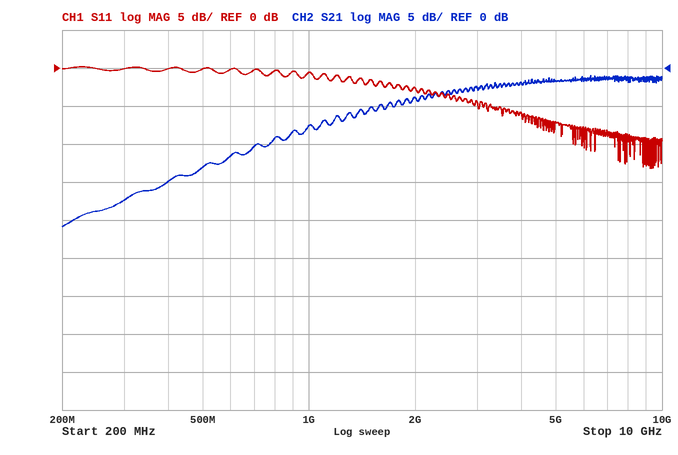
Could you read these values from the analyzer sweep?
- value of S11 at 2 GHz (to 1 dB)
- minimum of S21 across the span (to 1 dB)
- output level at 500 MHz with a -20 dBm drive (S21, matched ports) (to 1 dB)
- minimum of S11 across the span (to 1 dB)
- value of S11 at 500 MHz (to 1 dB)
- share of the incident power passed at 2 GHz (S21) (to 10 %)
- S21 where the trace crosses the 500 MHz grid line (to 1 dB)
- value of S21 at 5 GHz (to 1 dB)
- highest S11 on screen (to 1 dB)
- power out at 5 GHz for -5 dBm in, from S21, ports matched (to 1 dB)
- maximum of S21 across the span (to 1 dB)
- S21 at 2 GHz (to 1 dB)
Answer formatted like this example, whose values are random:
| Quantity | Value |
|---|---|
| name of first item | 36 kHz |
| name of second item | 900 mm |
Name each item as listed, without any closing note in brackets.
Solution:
| Quantity | Value |
|---|---|
| value of S11 at 2 GHz | -3 dB |
| minimum of S21 across the span | -21 dB |
| output level at 500 MHz with a -20 dBm drive (S21, matched ports) | -33 dBm |
| minimum of S11 across the span | -13 dB |
| value of S11 at 500 MHz | 0 dB |
| share of the incident power passed at 2 GHz (S21) | 40 % |
| S21 where the trace crosses the 500 MHz grid line | -13 dB |
| value of S21 at 5 GHz | -2 dB |
| highest S11 on screen | 0 dB |
| power out at 5 GHz for -5 dBm in, from S21, ports matched | -7 dBm |
| maximum of S21 across the span | -1 dB |
| S21 at 2 GHz | -4 dB |
